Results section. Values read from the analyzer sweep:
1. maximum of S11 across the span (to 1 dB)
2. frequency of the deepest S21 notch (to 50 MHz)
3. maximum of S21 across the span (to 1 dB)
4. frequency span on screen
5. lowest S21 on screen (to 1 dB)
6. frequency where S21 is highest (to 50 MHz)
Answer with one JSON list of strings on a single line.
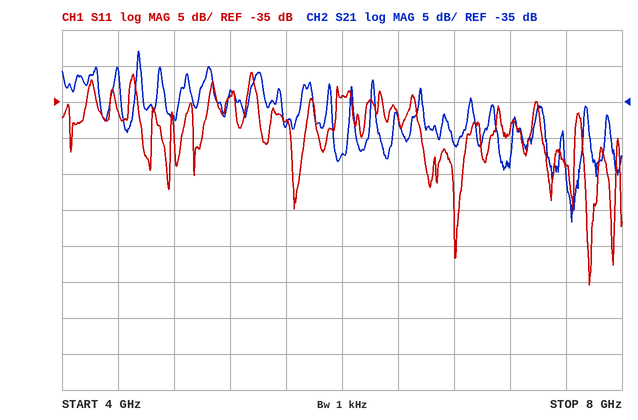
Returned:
["-31 dB", "7.65 GHz", "-28 dB", "4 GHz", "-52 dB", "4.55 GHz"]
